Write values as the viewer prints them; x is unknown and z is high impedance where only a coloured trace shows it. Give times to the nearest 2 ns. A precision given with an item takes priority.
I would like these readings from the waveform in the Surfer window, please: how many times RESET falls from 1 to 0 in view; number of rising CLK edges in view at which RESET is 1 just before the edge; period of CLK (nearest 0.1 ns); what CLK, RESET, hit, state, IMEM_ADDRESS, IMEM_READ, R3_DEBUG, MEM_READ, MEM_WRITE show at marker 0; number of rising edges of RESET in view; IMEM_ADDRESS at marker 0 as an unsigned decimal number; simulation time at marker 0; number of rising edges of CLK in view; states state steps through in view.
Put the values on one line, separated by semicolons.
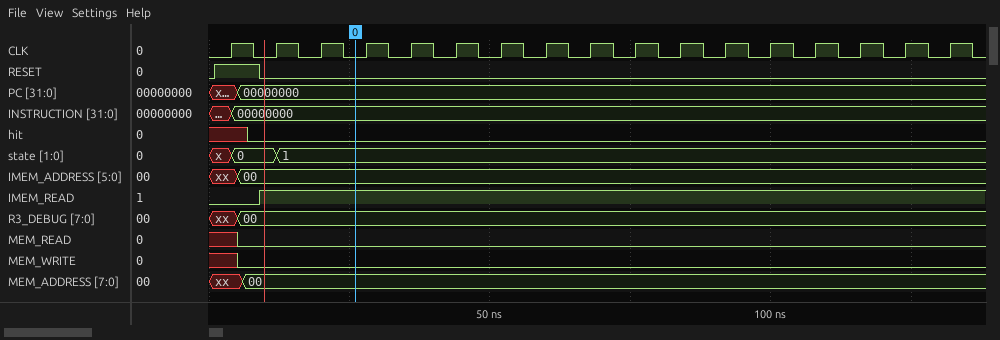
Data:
1; 1; 8 ns; CLK=0, RESET=0, hit=0, state=1, IMEM_ADDRESS=00, IMEM_READ=1, R3_DEBUG=00, MEM_READ=0, MEM_WRITE=0; 1; 0; 26 ns; 17; x, 0, 1
